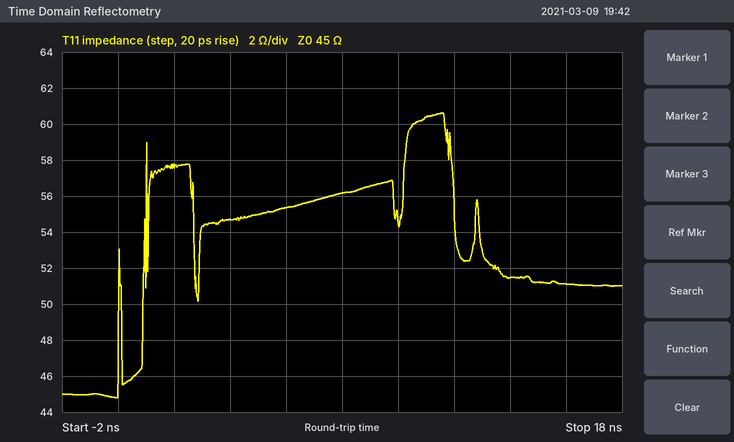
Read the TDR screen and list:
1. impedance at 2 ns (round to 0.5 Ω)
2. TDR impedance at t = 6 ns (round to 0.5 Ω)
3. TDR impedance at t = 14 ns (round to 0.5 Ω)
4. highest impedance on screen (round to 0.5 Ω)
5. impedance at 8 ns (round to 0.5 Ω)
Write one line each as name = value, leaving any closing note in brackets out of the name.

impedance at 2 ns = 57.5 Ω
TDR impedance at t = 6 ns = 55.5 Ω
TDR impedance at t = 14 ns = 51.5 Ω
highest impedance on screen = 60.5 Ω
impedance at 8 ns = 56.0 Ω
